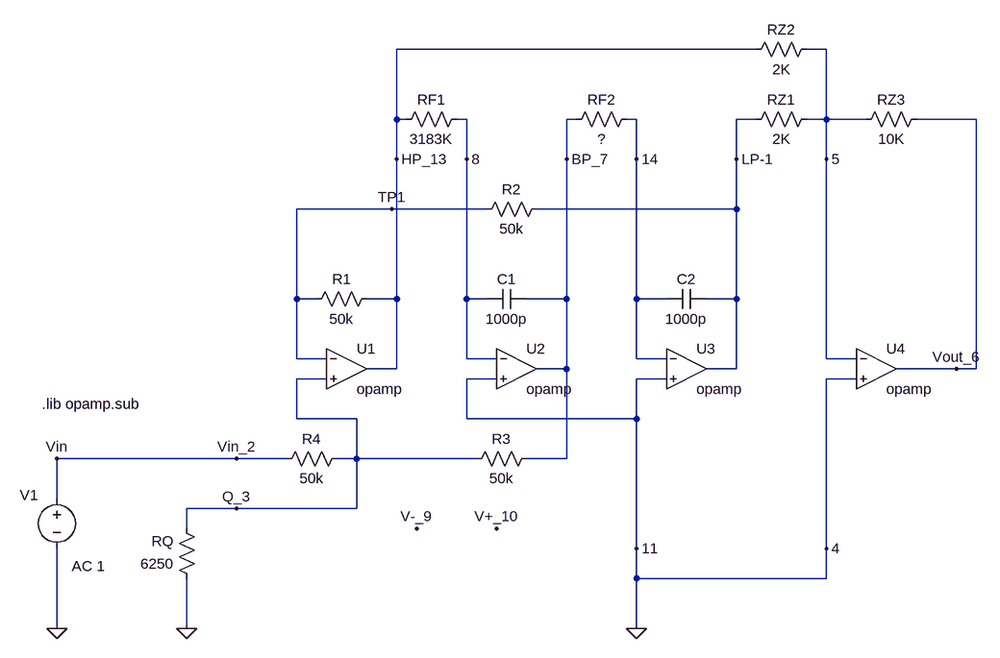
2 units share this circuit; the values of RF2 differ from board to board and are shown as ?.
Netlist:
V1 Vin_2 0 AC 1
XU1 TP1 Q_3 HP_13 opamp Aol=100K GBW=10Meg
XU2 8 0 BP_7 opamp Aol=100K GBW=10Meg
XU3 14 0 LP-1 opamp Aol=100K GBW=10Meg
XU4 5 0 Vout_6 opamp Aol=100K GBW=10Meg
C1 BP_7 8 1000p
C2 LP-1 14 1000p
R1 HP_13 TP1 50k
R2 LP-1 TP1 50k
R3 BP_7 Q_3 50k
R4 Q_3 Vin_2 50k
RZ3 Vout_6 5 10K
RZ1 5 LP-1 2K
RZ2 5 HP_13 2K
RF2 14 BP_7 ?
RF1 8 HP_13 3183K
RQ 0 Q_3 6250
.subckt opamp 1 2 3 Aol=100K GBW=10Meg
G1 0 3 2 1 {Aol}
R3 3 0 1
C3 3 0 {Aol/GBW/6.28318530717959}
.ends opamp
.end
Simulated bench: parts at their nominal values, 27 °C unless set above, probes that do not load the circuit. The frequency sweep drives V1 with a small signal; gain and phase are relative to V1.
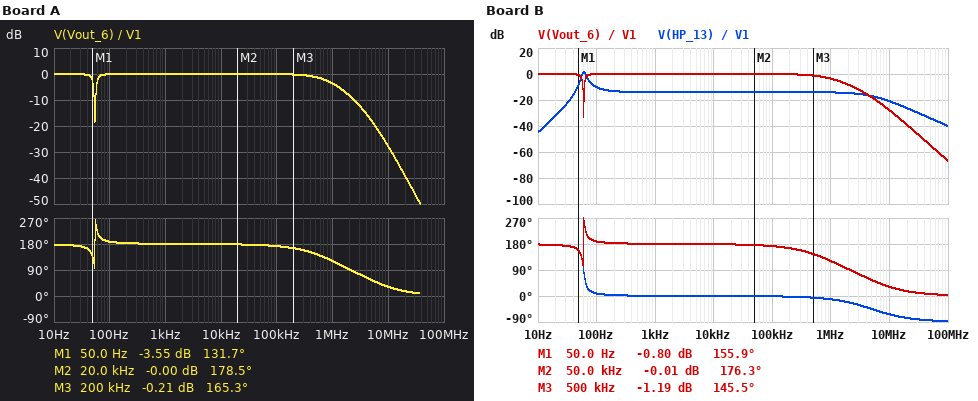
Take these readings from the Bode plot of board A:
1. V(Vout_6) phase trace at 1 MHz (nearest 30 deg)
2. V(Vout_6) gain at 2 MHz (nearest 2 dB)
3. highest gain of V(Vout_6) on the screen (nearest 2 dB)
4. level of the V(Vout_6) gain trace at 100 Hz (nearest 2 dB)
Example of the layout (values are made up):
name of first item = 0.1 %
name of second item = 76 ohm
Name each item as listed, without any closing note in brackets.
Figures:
V(Vout_6) phase trace at 1 MHz = 120 deg
V(Vout_6) gain at 2 MHz = -8 dB
highest gain of V(Vout_6) on the screen = 0 dB
level of the V(Vout_6) gain trace at 100 Hz = 0 dB
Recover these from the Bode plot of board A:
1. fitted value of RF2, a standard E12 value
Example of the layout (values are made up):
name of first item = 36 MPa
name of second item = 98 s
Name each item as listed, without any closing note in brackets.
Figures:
fitted value of RF2, a standard E12 value = 2.7 MΩ
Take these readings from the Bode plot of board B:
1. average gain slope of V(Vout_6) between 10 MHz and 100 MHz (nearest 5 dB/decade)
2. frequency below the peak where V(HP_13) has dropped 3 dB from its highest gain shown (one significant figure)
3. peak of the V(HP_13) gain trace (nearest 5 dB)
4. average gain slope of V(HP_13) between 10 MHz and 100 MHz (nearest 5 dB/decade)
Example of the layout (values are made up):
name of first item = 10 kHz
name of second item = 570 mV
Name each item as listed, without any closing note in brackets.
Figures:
average gain slope of V(Vout_6) between 10 MHz and 100 MHz = -40 dB/decade
frequency below the peak where V(HP_13) has dropped 3 dB from its highest gain shown = 60 Hz
peak of the V(HP_13) gain trace = 0 dB
average gain slope of V(HP_13) between 10 MHz and 100 MHz = -20 dB/decade
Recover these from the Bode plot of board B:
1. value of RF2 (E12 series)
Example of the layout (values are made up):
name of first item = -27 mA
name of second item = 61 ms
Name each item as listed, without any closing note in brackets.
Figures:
value of RF2 = 2.2 MΩ
